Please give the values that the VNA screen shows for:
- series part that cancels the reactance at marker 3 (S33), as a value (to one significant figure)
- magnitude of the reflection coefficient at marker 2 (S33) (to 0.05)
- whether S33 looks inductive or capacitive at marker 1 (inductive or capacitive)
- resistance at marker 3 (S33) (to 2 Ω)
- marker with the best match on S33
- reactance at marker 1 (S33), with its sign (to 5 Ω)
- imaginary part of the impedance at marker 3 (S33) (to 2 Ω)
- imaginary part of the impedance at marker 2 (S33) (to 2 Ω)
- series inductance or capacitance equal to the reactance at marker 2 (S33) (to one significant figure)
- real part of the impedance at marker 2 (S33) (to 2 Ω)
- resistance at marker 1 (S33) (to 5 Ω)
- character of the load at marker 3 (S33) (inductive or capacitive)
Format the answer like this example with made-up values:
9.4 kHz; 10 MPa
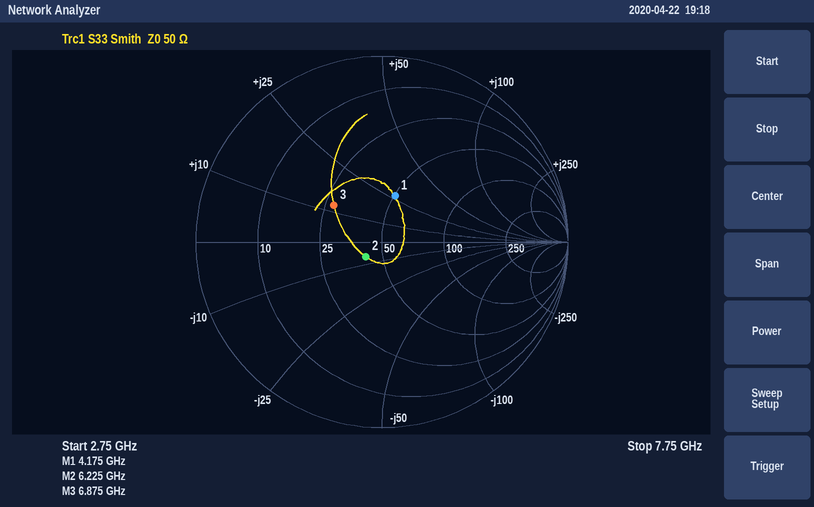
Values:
2 pF; 0.10; inductive; 28 Ω; marker 2; +25 Ω; +12 Ω; -6 Ω; 4 pF; 42 Ω; 50 Ω; inductive
